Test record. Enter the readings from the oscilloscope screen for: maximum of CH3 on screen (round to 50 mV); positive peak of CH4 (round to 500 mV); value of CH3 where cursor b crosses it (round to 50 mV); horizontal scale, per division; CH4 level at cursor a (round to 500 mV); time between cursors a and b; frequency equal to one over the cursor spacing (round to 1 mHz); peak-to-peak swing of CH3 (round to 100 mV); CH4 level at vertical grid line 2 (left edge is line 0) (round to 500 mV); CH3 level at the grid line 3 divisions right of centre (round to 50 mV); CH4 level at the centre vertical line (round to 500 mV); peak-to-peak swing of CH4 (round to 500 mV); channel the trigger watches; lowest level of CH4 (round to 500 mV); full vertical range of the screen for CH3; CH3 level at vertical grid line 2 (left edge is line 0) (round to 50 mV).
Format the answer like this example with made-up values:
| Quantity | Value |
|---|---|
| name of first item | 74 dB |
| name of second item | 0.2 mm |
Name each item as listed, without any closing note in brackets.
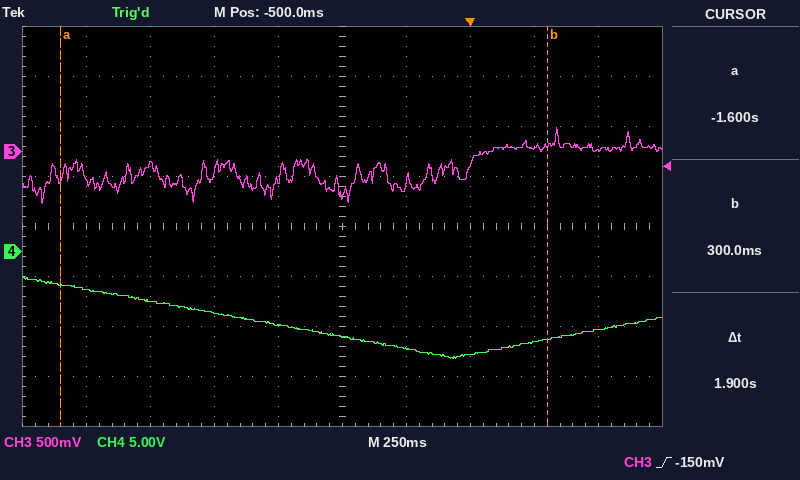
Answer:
| Quantity | Value |
|---|---|
| maximum of CH3 on screen | 250 mV |
| positive peak of CH4 | -2.5 V |
| value of CH3 where cursor b crosses it | 50 mV |
| horizontal scale, per division | 250 ms |
| CH4 level at cursor a | -3.5 V |
| time between cursors a and b | 1.9 s |
| frequency equal to one over the cursor spacing | 526 mHz |
| peak-to-peak swing of CH3 | 800 mV |
| CH4 level at vertical grid line 2 (left edge is line 0) | -5.0 V |
| CH3 level at the grid line 3 divisions right of centre | 50 mV |
| CH4 level at the centre vertical line | -8.5 V |
| peak-to-peak swing of CH4 | 8.0 V |
| channel the trigger watches | CH3 |
| lowest level of CH4 | -10.5 V |
| full vertical range of the screen for CH3 | 4 V |
| CH3 level at vertical grid line 2 (left edge is line 0) | -150 mV |
